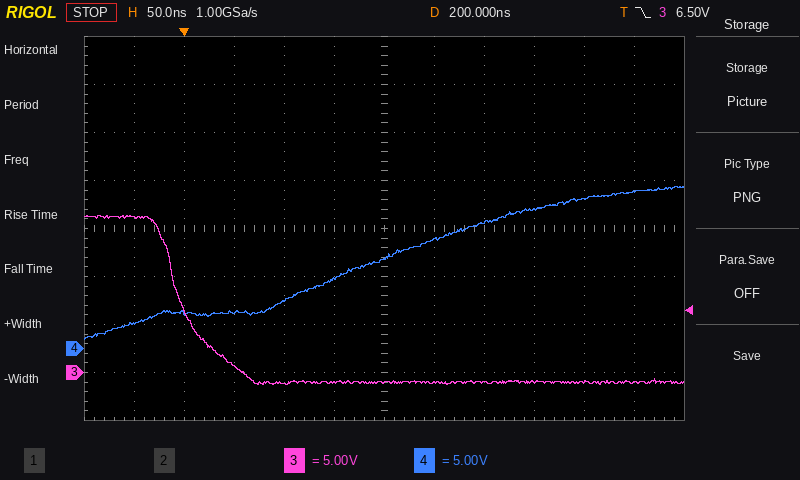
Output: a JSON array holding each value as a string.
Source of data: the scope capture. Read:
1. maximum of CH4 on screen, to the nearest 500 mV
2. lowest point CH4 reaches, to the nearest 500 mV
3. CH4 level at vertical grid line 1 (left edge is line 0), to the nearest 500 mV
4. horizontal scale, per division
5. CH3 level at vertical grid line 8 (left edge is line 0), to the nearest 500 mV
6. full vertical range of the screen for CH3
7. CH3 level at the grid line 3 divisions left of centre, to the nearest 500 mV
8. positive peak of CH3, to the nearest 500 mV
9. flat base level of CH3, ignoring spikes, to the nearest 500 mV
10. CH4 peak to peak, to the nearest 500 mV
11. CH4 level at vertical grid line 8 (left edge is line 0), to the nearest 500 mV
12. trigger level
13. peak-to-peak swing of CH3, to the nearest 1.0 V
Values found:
["17.0 V", "1.0 V", "2.5 V", "50 ns", "-1.0 V", "40 V", "500 mV", "16.5 V", "-1.0 V", "16.0 V", "13.0 V", "6.50 V", "18.0 V"]
